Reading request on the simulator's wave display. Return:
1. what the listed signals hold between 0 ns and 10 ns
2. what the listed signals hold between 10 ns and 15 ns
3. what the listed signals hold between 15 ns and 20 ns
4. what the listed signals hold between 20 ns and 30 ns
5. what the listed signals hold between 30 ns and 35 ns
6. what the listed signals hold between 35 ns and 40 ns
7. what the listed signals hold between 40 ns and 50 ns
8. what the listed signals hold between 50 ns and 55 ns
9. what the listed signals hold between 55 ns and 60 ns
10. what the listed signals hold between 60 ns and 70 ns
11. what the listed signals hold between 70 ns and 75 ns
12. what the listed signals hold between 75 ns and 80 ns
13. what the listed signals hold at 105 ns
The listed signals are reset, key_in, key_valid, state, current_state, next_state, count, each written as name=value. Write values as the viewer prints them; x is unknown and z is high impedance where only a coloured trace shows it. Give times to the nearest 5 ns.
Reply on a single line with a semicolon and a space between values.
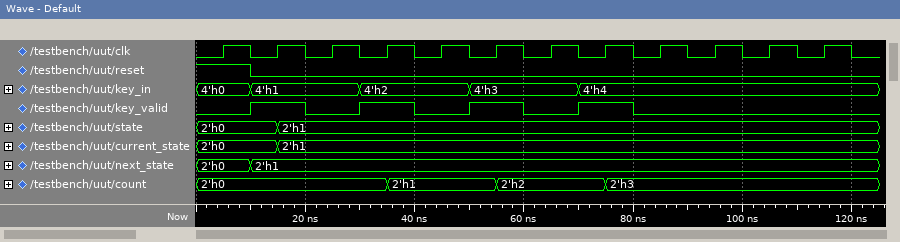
reset=1, key_in=4'h0, key_valid=0, state=2'h0, current_state=2'h0, next_state=2'h0, count=2'h0; reset=0, key_in=4'h1, key_valid=1, state=2'h0, current_state=2'h0, next_state=2'h1, count=2'h0; reset=0, key_in=4'h1, key_valid=1, state=2'h1, current_state=2'h1, next_state=2'h1, count=2'h0; reset=0, key_in=4'h1, key_valid=0, state=2'h1, current_state=2'h1, next_state=2'h1, count=2'h0; reset=0, key_in=4'h2, key_valid=1, state=2'h1, current_state=2'h1, next_state=2'h1, count=2'h0; reset=0, key_in=4'h2, key_valid=1, state=2'h1, current_state=2'h1, next_state=2'h1, count=2'h1; reset=0, key_in=4'h2, key_valid=0, state=2'h1, current_state=2'h1, next_state=2'h1, count=2'h1; reset=0, key_in=4'h3, key_valid=1, state=2'h1, current_state=2'h1, next_state=2'h1, count=2'h1; reset=0, key_in=4'h3, key_valid=1, state=2'h1, current_state=2'h1, next_state=2'h1, count=2'h2; reset=0, key_in=4'h3, key_valid=0, state=2'h1, current_state=2'h1, next_state=2'h1, count=2'h2; reset=0, key_in=4'h4, key_valid=1, state=2'h1, current_state=2'h1, next_state=2'h1, count=2'h2; reset=0, key_in=4'h4, key_valid=1, state=2'h1, current_state=2'h1, next_state=2'h1, count=2'h3; reset=0, key_in=4'h4, key_valid=0, state=2'h1, current_state=2'h1, next_state=2'h1, count=2'h3
